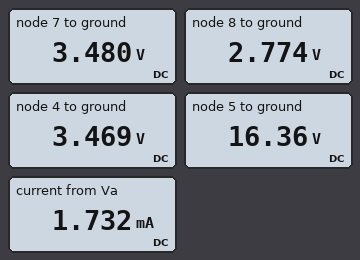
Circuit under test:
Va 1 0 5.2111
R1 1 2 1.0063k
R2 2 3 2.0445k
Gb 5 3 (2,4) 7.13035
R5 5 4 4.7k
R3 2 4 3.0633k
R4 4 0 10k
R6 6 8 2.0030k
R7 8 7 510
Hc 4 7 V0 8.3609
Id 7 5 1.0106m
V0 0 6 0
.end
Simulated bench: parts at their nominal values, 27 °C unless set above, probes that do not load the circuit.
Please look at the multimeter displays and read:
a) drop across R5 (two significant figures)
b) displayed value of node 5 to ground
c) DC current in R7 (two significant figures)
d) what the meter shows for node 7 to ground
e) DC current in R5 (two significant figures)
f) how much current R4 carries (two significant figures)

13 V
16.36 V
1.4 mA
3.480 V
2.7 mA
350 µA
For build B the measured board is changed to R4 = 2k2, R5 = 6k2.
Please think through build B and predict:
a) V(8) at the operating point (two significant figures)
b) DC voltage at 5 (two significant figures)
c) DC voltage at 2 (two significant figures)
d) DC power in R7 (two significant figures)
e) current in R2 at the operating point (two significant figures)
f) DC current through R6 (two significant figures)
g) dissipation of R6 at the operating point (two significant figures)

2.2 V
24 V
2.8 V
640 µW
2.4 mA
1.1 mA
2.5 mW
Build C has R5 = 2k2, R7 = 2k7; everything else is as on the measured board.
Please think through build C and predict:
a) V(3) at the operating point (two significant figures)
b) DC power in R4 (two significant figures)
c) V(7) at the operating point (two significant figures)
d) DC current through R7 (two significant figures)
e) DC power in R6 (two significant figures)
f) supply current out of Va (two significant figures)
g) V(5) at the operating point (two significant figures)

1.4 V
1.6 mW
4.0 V
840 µA
1.4 mW
1.2 mA
8.9 V
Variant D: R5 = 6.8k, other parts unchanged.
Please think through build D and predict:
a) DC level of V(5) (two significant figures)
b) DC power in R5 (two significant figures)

22 V
51 mW
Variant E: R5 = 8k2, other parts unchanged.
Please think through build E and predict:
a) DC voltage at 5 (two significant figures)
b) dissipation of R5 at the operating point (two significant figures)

26 V
62 mW
